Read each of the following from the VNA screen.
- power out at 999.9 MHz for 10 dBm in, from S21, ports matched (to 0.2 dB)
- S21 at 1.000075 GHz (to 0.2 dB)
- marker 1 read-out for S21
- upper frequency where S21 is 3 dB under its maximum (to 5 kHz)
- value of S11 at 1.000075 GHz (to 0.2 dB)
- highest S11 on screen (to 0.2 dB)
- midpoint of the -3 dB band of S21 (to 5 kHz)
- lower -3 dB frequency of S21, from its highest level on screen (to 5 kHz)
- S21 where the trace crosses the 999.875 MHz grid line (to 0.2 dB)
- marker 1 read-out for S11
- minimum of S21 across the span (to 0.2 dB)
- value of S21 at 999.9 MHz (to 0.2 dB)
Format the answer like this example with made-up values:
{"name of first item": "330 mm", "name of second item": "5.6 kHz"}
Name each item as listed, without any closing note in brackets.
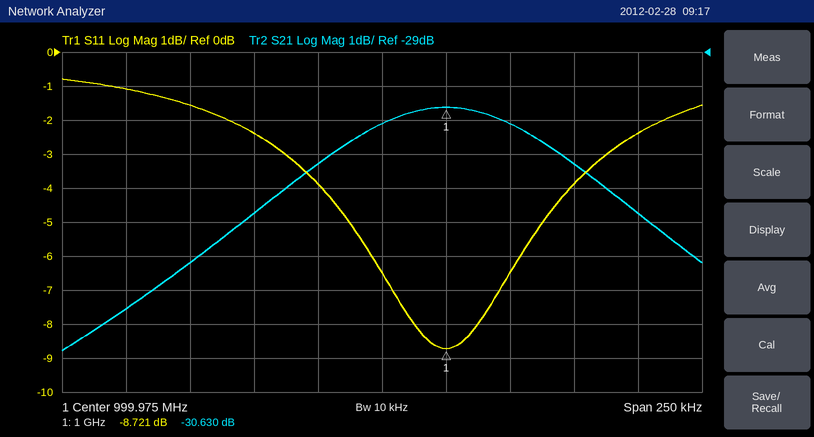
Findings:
{"power out at 999.9 MHz for 10 dBm in, from S21, ports matched": "-25.2 dBm", "S21 at 1.000075 GHz": "-33.8 dB", "marker 1 read-out for S21": "-30.630 dB", "upper frequency where S21 is 3 dB under its maximum": "1.000075 GHz", "value of S11 at 1.000075 GHz": "-2.4 dB", "highest S11 on screen": "-0.8 dB", "midpoint of the -3 dB band of S21": "1.000000 GHz", "lower -3 dB frequency of S21, from its highest level on screen": "999.925 MHz", "S21 where the trace crosses the 999.875 MHz grid line": "-36.6 dB", "marker 1 read-out for S11": "-8.721 dB", "minimum of S21 across the span": "-37.8 dB", "value of S21 at 999.9 MHz": "-35.2 dB"}
